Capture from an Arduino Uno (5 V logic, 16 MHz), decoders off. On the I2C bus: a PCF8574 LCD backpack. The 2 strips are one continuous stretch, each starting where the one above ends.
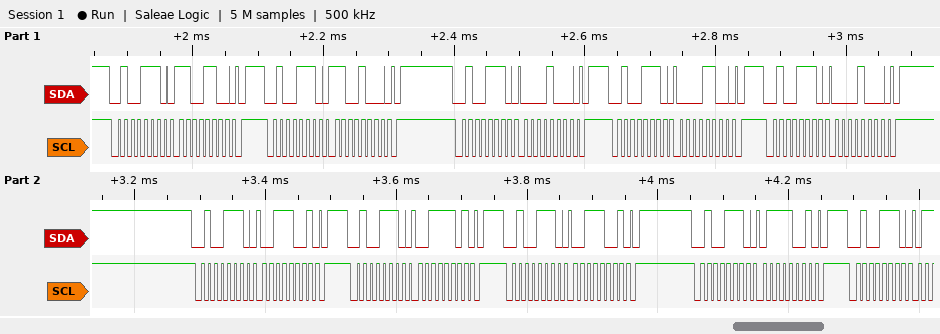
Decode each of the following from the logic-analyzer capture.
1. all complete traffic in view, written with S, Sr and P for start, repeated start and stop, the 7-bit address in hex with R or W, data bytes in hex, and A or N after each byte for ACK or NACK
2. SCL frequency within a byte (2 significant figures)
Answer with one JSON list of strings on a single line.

["S 27W A CC A P S 27W A C8 A P S 27W A 08 A P S 27W A 0C A P S 27W A 08 A P S 27W A 39 A P S 27W A 3D A P S 27W A 39 A P S 27W A 79 A P S 27W A", "100 kHz"]
